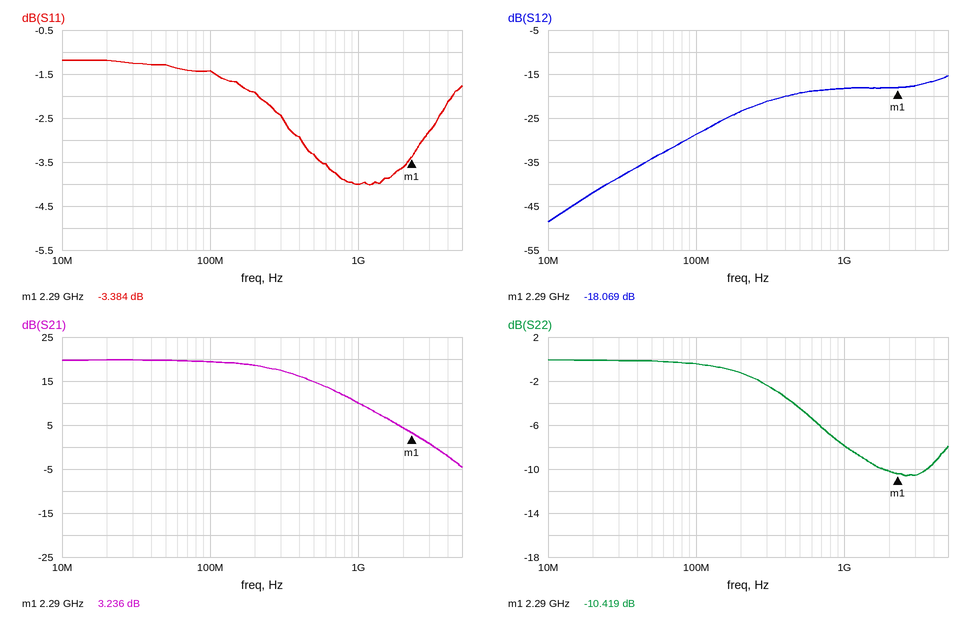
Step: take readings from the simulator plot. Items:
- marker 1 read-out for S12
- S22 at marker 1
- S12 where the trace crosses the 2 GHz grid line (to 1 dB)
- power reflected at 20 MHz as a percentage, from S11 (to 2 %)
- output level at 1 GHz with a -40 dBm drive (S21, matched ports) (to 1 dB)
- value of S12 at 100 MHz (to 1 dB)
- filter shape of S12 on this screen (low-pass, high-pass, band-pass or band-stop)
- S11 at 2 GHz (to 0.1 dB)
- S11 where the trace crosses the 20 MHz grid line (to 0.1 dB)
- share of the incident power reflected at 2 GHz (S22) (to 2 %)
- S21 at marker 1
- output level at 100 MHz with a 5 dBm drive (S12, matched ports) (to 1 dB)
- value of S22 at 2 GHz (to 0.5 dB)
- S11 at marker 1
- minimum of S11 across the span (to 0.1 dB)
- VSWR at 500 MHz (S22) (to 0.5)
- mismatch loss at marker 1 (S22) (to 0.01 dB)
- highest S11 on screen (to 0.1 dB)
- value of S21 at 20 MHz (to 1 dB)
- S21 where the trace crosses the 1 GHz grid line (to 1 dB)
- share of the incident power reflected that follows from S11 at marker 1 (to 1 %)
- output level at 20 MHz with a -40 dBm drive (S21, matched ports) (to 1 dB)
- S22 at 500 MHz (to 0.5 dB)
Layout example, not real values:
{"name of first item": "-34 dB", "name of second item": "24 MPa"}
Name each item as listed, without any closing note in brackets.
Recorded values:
{"marker 1 read-out for S12": "-18.069 dB", "S22 at marker 1": "-10.419 dB", "S12 where the trace crosses the 2 GHz grid line": "-18 dB", "power reflected at 20 MHz as a percentage, from S11": "76 %", "output level at 1 GHz with a -40 dBm drive (S21, matched ports)": "-30 dBm", "value of S12 at 100 MHz": "-29 dB", "filter shape of S12 on this screen": "high-pass", "S11 at 2 GHz": "-3.6 dB", "S11 where the trace crosses the 20 MHz grid line": "-1.2 dB", "share of the incident power reflected at 2 GHz (S22)": "10 %", "S21 at marker 1": "3.236 dB", "output level at 100 MHz with a 5 dBm drive (S12, matched ports)": "-24 dBm", "value of S22 at 2 GHz": "-10.0 dB", "S11 at marker 1": "-3.384 dB", "minimum of S11 across the span": "-4.0 dB", "VSWR at 500 MHz (S22)": "4.0", "mismatch loss at marker 1 (S22)": "0.41 dB", "highest S11 on screen": "-1.2 dB", "value of S21 at 20 MHz": "20 dB", "S21 where the trace crosses the 1 GHz grid line": "10 dB", "share of the incident power reflected that follows from S11 at marker 1": "46 %", "output level at 20 MHz with a -40 dBm drive (S21, matched ports)": "-20 dBm", "S22 at 500 MHz": "-4.5 dB"}
